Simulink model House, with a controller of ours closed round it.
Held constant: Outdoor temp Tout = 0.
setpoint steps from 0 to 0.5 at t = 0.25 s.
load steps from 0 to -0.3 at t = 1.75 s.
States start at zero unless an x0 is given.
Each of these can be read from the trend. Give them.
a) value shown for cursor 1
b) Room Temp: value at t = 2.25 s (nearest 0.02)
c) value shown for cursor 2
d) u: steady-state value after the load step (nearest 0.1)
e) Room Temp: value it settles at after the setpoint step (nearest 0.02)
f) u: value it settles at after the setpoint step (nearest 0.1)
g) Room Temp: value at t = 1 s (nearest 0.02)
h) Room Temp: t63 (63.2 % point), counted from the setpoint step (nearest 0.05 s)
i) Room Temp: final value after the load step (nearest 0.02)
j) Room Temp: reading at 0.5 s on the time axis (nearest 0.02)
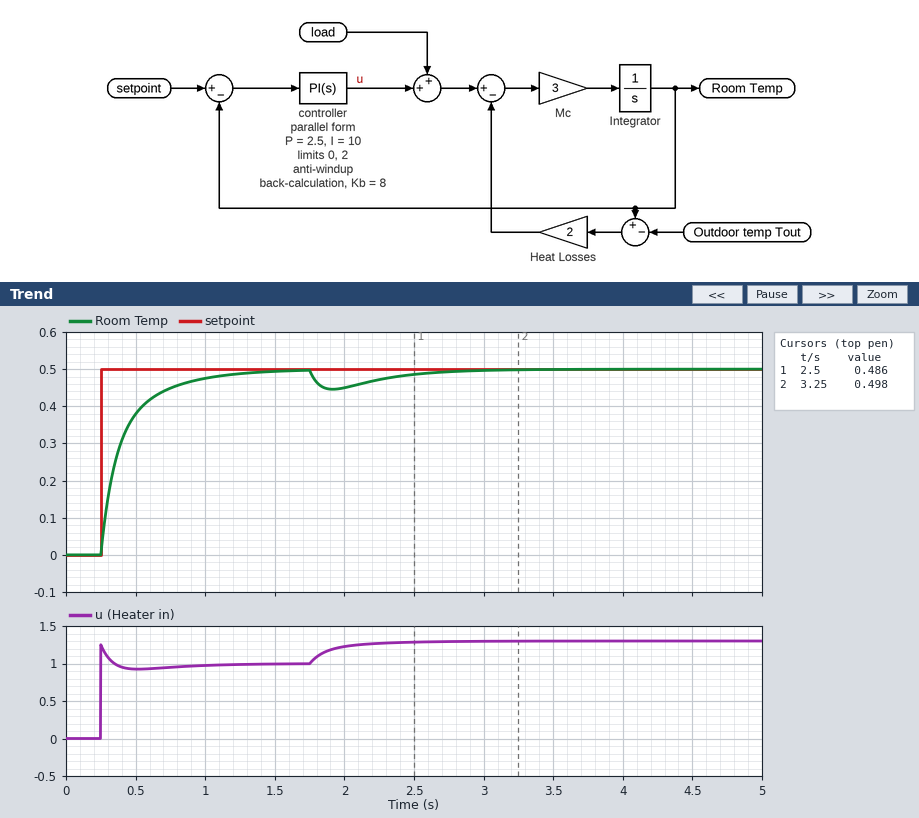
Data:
0.486
0.48
0.498
1.3
0.50
1.0
0.48
0.15 s
0.50
0.38
